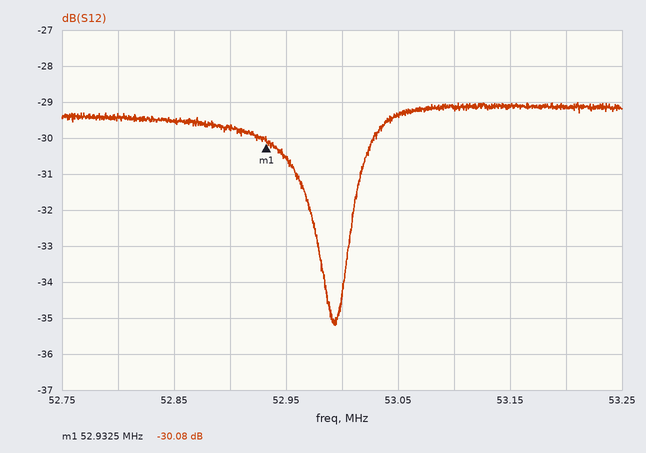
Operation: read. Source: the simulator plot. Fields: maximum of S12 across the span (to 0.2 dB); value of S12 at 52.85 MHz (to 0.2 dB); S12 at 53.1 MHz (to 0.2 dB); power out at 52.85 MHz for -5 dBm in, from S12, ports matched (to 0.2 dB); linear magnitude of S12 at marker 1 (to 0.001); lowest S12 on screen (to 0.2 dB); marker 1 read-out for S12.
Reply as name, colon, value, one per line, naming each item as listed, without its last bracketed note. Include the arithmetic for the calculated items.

maximum of S12 across the span: -29.0 dB
value of S12 at 52.85 MHz: -29.6 dB
S12 at 53.1 MHz: -29.2 dB
power out at 52.85 MHz for -5 dBm in, from S12, ports matched: -5 dBm + (-29.6 dB) = -34.6 dBm
linear magnitude of S12 at marker 1: 10^(-30.08/20) ≈ 0.031
lowest S12 on screen: -35.2 dB
marker 1 read-out for S12: -30.08 dB
